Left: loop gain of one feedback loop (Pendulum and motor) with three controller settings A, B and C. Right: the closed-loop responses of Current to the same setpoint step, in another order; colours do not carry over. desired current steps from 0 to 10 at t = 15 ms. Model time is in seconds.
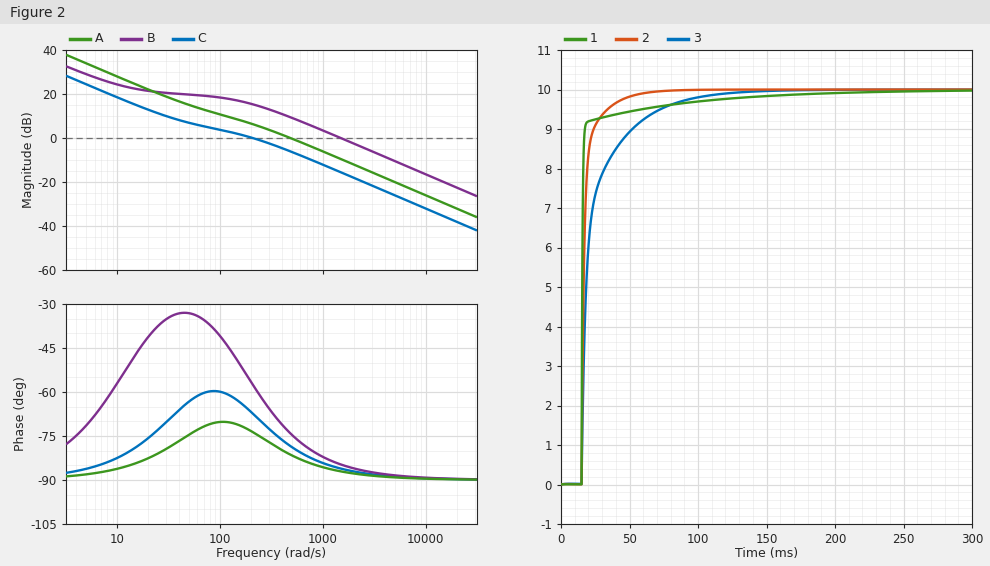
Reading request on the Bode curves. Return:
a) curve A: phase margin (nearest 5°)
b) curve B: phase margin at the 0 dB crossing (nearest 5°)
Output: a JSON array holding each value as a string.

["100°", "95°"]
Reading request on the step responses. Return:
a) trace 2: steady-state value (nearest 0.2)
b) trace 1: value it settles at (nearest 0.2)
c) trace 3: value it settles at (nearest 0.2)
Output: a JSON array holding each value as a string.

["10.0", "10.0", "10.0"]
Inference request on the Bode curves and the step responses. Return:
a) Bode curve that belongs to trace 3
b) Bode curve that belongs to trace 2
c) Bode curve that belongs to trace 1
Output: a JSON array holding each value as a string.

["C", "A", "B"]
